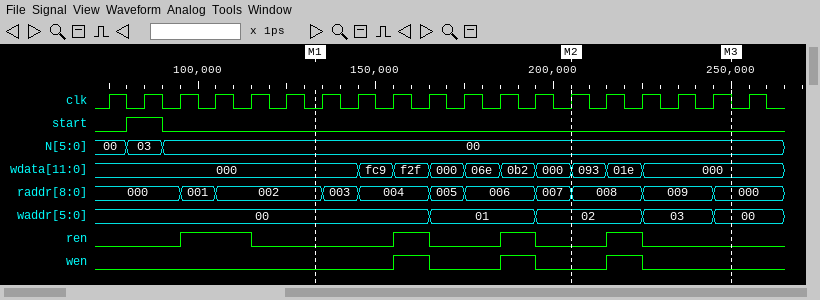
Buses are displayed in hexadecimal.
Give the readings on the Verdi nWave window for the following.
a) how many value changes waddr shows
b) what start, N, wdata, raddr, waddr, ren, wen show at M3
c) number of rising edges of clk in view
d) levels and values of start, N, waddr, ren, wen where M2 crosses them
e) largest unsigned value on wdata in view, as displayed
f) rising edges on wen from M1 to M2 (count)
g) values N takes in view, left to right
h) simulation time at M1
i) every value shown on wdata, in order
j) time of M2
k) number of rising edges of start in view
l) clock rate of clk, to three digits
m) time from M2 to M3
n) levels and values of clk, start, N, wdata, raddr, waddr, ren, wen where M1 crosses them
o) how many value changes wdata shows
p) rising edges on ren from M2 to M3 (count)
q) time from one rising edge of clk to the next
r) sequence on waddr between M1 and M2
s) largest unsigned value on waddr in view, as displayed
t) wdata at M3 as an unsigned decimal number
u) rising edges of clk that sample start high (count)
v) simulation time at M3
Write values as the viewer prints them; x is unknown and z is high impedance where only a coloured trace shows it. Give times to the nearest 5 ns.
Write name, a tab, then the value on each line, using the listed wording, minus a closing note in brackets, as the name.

how many value changes waddr shows	4
what start, N, wdata, raddr, waddr, ren, wen show at M3	start=0, N=00, wdata=000, raddr=000, waddr=00, ren=0, wen=0
number of rising edges of clk in view	19
levels and values of start, N, waddr, ren, wen where M2 crosses them	start=0, N=00, waddr=02, ren=0, wen=0
largest unsigned value on wdata in view, as displayed	fc9
rising edges on wen from M1 to M2	2
values N takes in view, left to right	00, 03, 00
simulation time at M1	135 ns
every value shown on wdata, in order	000, fc9, f2f, 000, 06e, 0b2, 000, 093, 01e, 000
time of M2	205 ns
number of rising edges of start in view	1
clock rate of clk, to three digits	100 MHz
time from M2 to M3	45 ns
levels and values of clk, start, N, wdata, raddr, waddr, ren, wen where M1 crosses them	clk=0, start=0, N=00, wdata=000, raddr=002, waddr=00, ren=0, wen=0
how many value changes wdata shows	9
rising edges on ren from M2 to M3	1
time from one rising edge of clk to the next	10 ns
sequence on waddr between M1 and M2	00, 01, 02
largest unsigned value on waddr in view, as displayed	03
wdata at M3 as an unsigned decimal number	0
rising edges of clk that sample start high	1
simulation time at M3	250 ns
